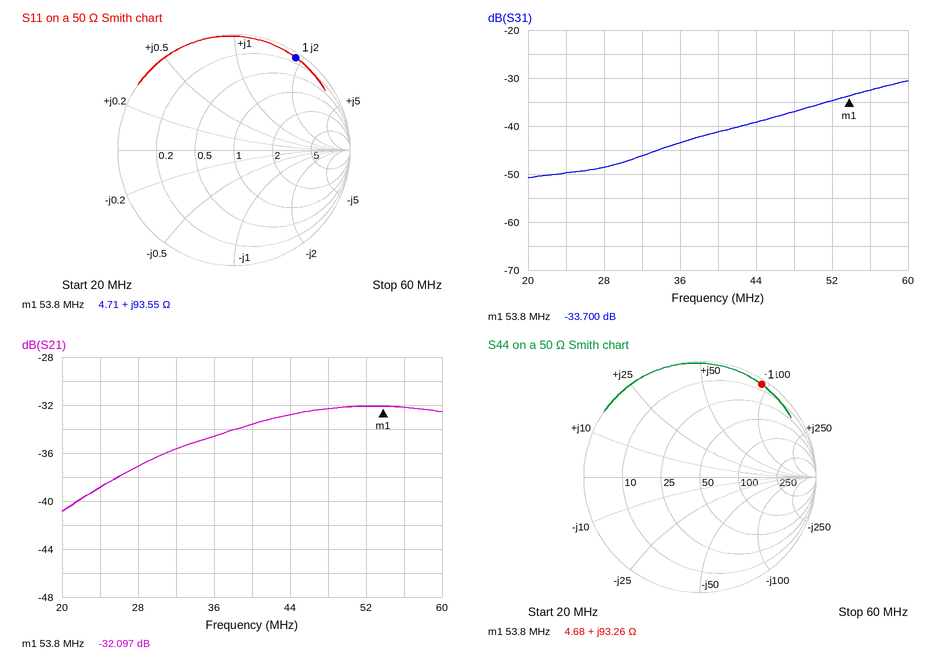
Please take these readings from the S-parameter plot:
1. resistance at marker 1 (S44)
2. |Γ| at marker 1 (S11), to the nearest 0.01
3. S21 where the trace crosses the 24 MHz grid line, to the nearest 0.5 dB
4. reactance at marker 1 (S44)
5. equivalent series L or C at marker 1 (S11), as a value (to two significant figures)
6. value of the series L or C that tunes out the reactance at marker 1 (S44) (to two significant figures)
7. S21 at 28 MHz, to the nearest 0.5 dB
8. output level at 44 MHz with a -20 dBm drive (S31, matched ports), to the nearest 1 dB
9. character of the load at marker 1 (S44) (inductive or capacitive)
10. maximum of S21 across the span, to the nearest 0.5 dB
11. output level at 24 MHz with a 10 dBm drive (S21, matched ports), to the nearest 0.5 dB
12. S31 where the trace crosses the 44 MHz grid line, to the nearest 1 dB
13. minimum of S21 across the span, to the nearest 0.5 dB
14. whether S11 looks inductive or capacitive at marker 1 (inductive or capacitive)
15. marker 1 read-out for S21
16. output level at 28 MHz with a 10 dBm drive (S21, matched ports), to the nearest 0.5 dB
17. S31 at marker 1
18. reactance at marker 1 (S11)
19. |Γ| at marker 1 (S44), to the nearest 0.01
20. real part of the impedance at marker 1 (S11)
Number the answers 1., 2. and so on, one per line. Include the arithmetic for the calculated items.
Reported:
1. 4.68 Ω
2. 0.96
3. -39.0 dB
4. +93.26 Ω
5. L = 93.55 Ω/(2π × 53.8 MHz) ≈ 277 nH, so 280 nH to two significant figures
6. C = 1/(2π × 53.8 MHz × 93.26 Ω) ≈ 32 pF
7. -37.0 dB
8. -20 dBm + (-39 dB) = -59 dBm
9. inductive
10. -32.0 dB
11. 10 dBm + (-39.0 dB) = -29.0 dBm
12. -39 dB
13. -41.0 dB
14. inductive
15. -32.097 dB
16. 10 dBm + (-37.0 dB) = -27.0 dBm
17. -33.700 dB
18. +93.55 Ω
19. 0.96
20. 4.71 Ω
